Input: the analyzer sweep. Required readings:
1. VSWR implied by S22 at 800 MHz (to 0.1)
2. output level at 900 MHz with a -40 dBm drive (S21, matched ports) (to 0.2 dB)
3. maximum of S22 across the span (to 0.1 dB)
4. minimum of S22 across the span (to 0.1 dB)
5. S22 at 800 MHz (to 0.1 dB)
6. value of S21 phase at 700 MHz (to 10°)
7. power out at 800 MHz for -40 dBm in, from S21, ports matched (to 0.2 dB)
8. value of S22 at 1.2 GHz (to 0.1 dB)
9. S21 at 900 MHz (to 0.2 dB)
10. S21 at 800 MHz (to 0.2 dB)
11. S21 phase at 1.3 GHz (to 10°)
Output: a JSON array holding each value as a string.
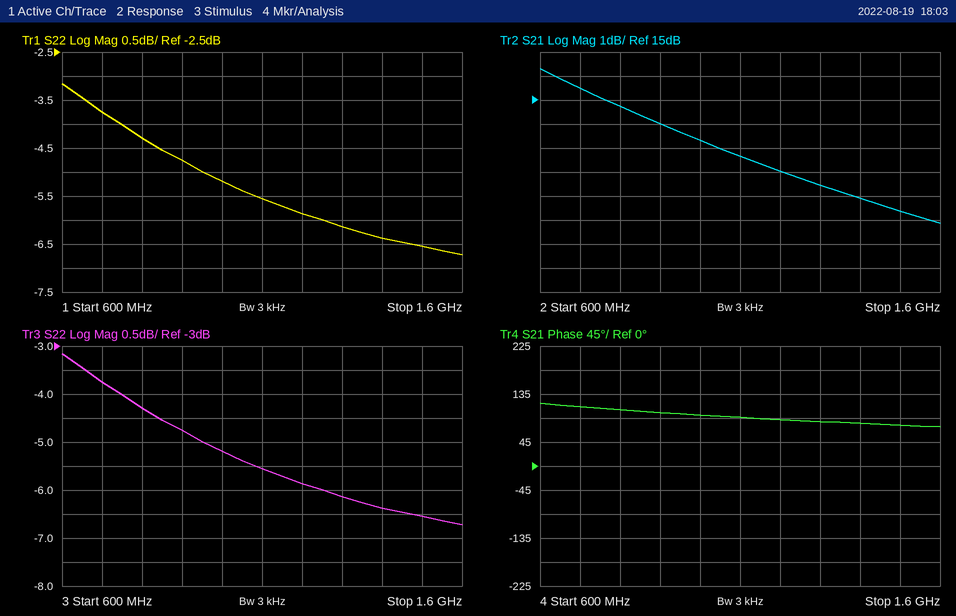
["4.1", "-26.0 dBm", "-3.2 dB", "-6.7 dB", "-4.3 dB", "110°", "-25.2 dBm", "-5.9 dB", "14.0 dB", "14.8 dB", "80°"]
